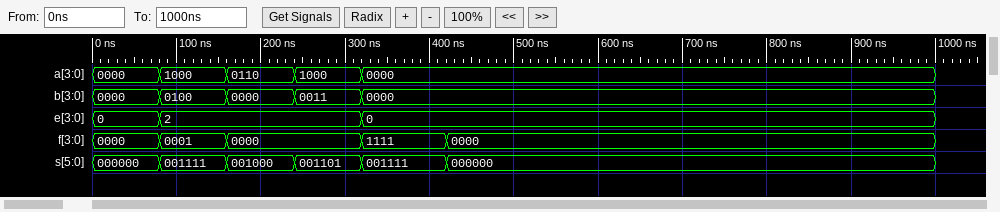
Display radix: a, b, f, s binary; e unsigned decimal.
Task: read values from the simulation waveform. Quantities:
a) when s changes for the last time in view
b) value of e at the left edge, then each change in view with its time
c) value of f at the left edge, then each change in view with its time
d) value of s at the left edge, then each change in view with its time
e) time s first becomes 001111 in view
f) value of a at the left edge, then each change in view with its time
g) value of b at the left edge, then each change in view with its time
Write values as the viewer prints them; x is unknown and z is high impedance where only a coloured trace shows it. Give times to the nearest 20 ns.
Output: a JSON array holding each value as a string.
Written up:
["420 ns", "0, 2 at 80 ns, 0 at 320 ns", "0000, 0001 at 80 ns, 0000 at 160 ns, 1111 at 320 ns, 0000 at 420 ns", "000000, 001111 at 80 ns, 001000 at 160 ns, 001101 at 240 ns, 001111 at 320 ns, 000000 at 420 ns", "80 ns", "0000, 1000 at 80 ns, 0110 at 160 ns, 1000 at 240 ns, 0000 at 320 ns", "0000, 0100 at 80 ns, 0000 at 160 ns, 0011 at 240 ns, 0000 at 320 ns"]
